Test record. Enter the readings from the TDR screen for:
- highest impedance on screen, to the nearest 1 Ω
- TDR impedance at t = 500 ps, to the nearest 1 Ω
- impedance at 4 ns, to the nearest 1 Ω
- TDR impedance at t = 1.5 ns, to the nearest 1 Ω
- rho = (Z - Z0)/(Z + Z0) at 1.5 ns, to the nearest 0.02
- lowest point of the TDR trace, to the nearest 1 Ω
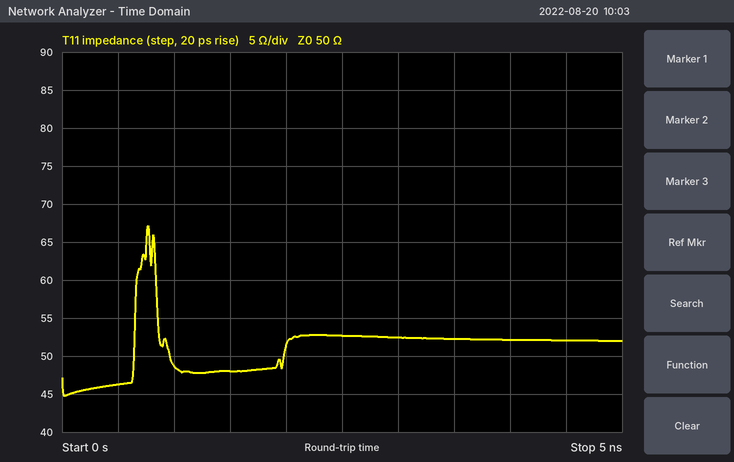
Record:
67 Ω
46 Ω
52 Ω
48 Ω
-0.02
45 Ω
